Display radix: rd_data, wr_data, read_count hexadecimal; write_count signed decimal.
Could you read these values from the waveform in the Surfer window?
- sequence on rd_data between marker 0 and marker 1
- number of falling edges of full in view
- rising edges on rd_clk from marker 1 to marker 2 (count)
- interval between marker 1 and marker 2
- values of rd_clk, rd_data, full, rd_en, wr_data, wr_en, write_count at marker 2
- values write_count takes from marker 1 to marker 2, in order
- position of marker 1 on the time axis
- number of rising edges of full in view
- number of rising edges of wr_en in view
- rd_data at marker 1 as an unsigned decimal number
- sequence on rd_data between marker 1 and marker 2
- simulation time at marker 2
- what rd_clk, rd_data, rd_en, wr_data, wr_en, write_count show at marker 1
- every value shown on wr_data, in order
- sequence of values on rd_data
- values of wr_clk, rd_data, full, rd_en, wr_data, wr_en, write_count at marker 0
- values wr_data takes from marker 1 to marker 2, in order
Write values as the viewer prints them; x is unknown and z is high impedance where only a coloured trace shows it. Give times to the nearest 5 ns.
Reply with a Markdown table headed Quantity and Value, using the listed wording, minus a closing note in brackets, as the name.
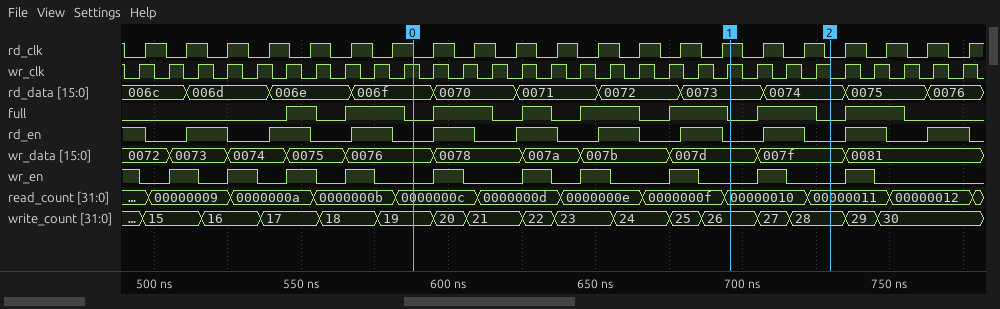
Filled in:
| Quantity | Value |
|---|---|
| sequence on rd_data between marker 0 and marker 1 | 006f, 0070, 0071, 0072, 0073 |
| number of falling edges of full in view | 8 |
| rising edges on rd_clk from marker 1 to marker 2 | 2 |
| interval between marker 1 and marker 2 | 35 ns |
| values of rd_clk, rd_data, full, rd_en, wr_data, wr_en, write_count at marker 2 | rd_clk=0, rd_data=0074, full=0, rd_en=0, wr_data=007f, wr_en=0, write_count=28 |
| values write_count takes from marker 1 to marker 2, in order | 26, 27, 28 |
| position of marker 1 on the time axis | 695 ns |
| number of rising edges of full in view | 8 |
| number of rising edges of wr_en in view | 10 |
| rd_data at marker 1 as an unsigned decimal number | 115 |
| sequence on rd_data between marker 1 and marker 2 | 0073, 0074 |
| simulation time at marker 2 | 730 ns |
| what rd_clk, rd_data, rd_en, wr_data, wr_en, write_count show at marker 1 | rd_clk=1, rd_data=0073, rd_en=0, wr_data=007d, wr_en=0, write_count=26 |
| every value shown on wr_data, in order | 0072, 0073, 0074, 0075, 0076, 0078, 007a, 007b, 007d, 007f, 0081 |
| sequence of values on rd_data | 006c, 006d, 006e, 006f, 0070, 0071, 0072, 0073, 0074, 0075, 0076 |
| values of wr_clk, rd_data, full, rd_en, wr_data, wr_en, write_count at marker 0 | wr_clk=1, rd_data=006f, full=0, rd_en=0, wr_data=0076, wr_en=0, write_count=19 |
| values wr_data takes from marker 1 to marker 2, in order | 007d, 007f |
